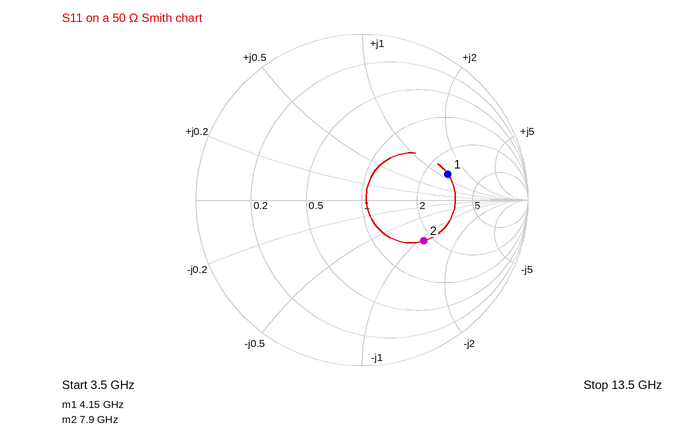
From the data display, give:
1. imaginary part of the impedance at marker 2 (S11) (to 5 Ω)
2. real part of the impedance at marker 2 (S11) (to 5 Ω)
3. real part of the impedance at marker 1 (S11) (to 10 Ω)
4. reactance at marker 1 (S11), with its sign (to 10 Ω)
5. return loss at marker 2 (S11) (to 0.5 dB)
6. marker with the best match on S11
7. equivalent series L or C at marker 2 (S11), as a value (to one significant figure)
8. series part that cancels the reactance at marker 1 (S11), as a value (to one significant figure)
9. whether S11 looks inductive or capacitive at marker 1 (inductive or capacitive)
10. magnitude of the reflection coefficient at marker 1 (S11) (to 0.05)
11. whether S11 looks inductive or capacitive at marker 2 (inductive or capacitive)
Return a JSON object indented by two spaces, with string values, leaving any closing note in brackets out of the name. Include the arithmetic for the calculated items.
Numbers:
{
  "imaginary part of the impedance at marker 2 (S11)": "-55 Ω",
  "real part of the impedance at marker 2 (S11)": "90 Ω",
  "real part of the impedance at marker 1 (S11)": "140 Ω",
  "reactance at marker 1 (S11), with its sign": "+60 Ω",
  "return loss at marker 2 (S11)": "7.0 dB",
  "marker with the best match on S11": "marker 2",
  "equivalent series L or C at marker 2 (S11), as a value": "C = 1/(2π × 7.9 GHz × 55 Ω) ≈ 366 fF, so 400 fF to one significant figure",
  "series part that cancels the reactance at marker 1 (S11), as a value": "C = 1/(2π × 4.15 GHz × 60 Ω) ≈ 639 fF, so 600 fF to one significant figure",
  "whether S11 looks inductive or capacitive at marker 1": "inductive",
  "magnitude of the reflection coefficient at marker 1 (S11)": "0.55",
  "whether S11 looks inductive or capacitive at marker 2": "capacitive"
}
